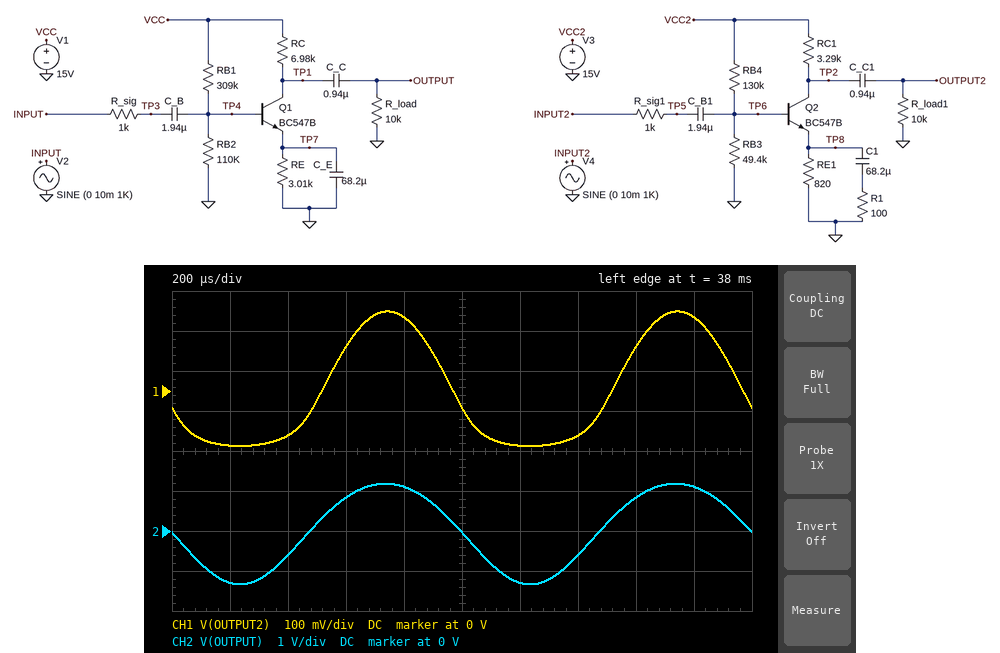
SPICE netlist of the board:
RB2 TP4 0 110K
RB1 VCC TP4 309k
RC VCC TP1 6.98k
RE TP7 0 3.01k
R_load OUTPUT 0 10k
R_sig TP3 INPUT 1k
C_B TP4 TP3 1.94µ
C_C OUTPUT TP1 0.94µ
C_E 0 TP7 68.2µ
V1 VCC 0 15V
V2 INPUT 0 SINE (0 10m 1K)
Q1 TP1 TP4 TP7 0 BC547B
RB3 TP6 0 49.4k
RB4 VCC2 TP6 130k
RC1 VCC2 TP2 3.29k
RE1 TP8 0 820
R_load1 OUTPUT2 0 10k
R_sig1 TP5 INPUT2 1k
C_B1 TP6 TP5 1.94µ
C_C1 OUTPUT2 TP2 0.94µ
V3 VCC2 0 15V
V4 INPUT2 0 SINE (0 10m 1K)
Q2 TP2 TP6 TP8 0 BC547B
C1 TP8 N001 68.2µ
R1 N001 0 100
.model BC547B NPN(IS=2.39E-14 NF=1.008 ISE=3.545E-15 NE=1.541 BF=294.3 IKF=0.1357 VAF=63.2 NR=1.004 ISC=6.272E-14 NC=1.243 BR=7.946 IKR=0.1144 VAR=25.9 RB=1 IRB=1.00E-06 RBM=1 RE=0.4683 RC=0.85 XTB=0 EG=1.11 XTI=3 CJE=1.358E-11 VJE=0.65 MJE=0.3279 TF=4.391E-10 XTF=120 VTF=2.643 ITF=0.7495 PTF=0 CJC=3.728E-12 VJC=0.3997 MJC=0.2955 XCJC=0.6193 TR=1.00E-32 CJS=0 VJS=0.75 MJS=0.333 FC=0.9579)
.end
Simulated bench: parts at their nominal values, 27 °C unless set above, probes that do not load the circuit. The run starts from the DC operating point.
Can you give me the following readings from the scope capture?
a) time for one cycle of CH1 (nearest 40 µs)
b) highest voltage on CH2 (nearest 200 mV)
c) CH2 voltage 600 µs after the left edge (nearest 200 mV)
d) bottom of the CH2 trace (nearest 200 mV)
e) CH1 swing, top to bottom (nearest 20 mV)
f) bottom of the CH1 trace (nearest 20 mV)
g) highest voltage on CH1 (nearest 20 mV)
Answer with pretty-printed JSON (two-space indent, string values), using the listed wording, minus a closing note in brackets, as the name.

{
  "time for one cycle of CH1": "1.00 ms",
  "highest voltage on CH2": "1.2 V",
  "CH2 voltage 600 µs after the left edge": "800 mV",
  "bottom of the CH2 trace": "-1.4 V",
  "CH1 swing, top to bottom": "340 mV",
  "bottom of the CH1 trace": "-140 mV",
  "highest voltage on CH1": "200 mV"
}
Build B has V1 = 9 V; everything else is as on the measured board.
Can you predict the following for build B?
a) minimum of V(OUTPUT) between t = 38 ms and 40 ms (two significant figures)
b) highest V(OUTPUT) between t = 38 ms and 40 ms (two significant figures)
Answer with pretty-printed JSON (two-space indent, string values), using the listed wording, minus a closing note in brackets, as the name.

{
  "minimum of V(OUTPUT) between t = 38 ms and 40 ms": "-780 mV",
  "highest V(OUTPUT) between t = 38 ms and 40 ms": "670 mV"
}
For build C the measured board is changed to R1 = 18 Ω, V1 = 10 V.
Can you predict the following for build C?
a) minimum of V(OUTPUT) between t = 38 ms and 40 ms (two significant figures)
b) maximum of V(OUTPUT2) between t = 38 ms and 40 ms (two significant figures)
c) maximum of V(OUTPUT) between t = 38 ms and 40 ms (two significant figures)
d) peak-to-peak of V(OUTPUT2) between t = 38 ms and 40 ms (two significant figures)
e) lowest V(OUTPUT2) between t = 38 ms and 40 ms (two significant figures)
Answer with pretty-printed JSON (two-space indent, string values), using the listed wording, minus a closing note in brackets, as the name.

{
  "minimum of V(OUTPUT) between t = 38 ms and 40 ms": "-880 mV",
  "maximum of V(OUTPUT2) between t = 38 ms and 40 ms": "560 mV",
  "maximum of V(OUTPUT) between t = 38 ms and 40 ms": "760 mV",
  "peak-to-peak of V(OUTPUT2) between t = 38 ms and 40 ms": "860 mV",
  "lowest V(OUTPUT2) between t = 38 ms and 40 ms": "-300 mV"
}
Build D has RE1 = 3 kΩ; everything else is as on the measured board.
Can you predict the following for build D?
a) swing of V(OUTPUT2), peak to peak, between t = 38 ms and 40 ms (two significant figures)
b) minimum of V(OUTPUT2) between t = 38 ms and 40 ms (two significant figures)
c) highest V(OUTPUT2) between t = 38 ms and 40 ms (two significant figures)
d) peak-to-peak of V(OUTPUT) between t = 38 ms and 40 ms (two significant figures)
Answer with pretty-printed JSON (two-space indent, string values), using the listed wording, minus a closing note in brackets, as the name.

{
  "swing of V(OUTPUT2), peak to peak, between t = 38 ms and 40 ms": "380 mV",
  "minimum of V(OUTPUT2) between t = 38 ms and 40 ms": "-190 mV",
  "highest V(OUTPUT2) between t = 38 ms and 40 ms": "190 mV",
  "peak-to-peak of V(OUTPUT) between t = 38 ms and 40 ms": "2.5 V"
}
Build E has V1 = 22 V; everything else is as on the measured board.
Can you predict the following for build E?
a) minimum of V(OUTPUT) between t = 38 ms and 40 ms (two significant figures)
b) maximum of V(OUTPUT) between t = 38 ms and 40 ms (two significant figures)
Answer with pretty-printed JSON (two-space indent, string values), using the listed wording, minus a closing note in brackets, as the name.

{
  "minimum of V(OUTPUT) between t = 38 ms and 40 ms": "-1.9 V",
  "maximum of V(OUTPUT) between t = 38 ms and 40 ms": "1.7 V"
}
